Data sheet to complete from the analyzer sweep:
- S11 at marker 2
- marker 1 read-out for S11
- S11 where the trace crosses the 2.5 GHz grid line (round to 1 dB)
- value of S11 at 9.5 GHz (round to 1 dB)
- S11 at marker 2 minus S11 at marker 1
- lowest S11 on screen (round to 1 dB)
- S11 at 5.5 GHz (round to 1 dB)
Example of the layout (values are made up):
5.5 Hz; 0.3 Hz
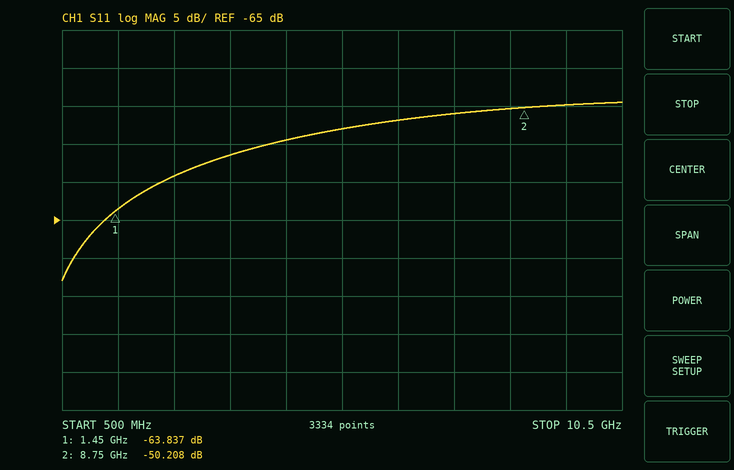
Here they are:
-50.208 dB; -63.837 dB; -59 dB; -50 dB; 13.629 dB; -73 dB; -53 dB
